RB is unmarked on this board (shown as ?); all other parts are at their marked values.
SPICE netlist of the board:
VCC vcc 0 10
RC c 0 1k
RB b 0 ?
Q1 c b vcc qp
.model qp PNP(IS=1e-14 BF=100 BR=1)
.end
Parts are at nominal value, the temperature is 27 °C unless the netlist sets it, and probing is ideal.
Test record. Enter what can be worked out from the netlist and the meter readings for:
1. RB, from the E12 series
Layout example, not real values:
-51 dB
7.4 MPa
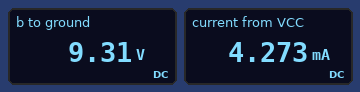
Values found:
220 kΩ
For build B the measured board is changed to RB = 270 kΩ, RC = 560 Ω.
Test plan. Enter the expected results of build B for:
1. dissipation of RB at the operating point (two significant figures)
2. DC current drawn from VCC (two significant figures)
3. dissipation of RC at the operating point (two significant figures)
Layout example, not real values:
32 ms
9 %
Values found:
320 µW
3.5 mA
6.7 mW
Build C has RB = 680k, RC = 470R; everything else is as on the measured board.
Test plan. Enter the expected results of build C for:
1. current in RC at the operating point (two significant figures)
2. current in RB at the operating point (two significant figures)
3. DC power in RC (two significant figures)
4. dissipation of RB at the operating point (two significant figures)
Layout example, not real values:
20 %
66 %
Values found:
1.4 mA
14 µA
890 µW
130 µW
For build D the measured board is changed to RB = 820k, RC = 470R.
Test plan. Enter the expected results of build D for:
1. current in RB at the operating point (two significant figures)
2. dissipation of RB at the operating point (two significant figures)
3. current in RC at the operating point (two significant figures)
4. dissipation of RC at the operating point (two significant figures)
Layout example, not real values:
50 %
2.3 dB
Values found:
11 µA
110 µW
1.1 mA
610 µW
